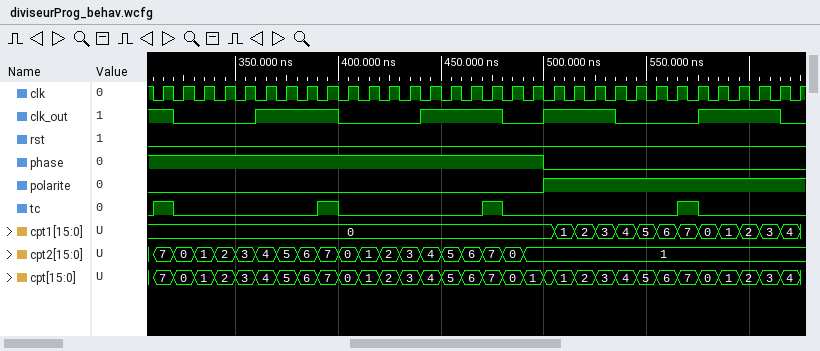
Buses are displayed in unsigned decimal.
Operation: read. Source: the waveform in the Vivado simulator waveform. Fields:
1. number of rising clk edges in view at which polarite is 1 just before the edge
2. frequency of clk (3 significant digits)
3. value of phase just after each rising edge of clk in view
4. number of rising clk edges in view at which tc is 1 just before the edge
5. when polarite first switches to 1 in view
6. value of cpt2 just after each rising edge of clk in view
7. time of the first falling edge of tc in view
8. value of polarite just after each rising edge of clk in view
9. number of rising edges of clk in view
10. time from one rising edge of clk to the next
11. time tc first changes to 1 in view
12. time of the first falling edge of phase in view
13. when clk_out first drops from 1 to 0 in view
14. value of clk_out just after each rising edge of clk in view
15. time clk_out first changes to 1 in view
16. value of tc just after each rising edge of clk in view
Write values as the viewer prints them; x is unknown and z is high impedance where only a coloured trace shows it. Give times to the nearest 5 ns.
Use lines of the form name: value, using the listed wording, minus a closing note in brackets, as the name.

number of rising clk edges in view at which polarite is 1 just before the edge: 13
frequency of clk: 100 MHz
value of phase just after each rising edge of clk in view: 1 1 1 1 1 1 1 1 1 1 1 1 1 1 1 1 1 1 1 0 0 0 0 0 0 0 0 0 0 0 0 0
number of rising clk edges in view at which tc is 1 just before the edge: 4
when polarite first switches to 1 in view: 500 ns
value of cpt2 just after each rising edge of clk in view: 7, 0, 1, 2, 3, 4, 5, 6, 7, 0, 1, 2, 3, 4, 5, 6, 7, 0, 1, 1, 1, 1, 1, 1, 1, 1, 1, 1, 1, 1, 1, 1
time of the first falling edge of tc in view: 320 ns
value of polarite just after each rising edge of clk in view: 0 0 0 0 0 0 0 0 0 0 0 0 0 0 0 0 0 0 0 1 1 1 1 1 1 1 1 1 1 1 1 1
number of rising edges of clk in view: 32
time from one rising edge of clk to the next: 10 ns
time tc first changes to 1 in view: 310 ns
time of the first falling edge of phase in view: 500 ns
when clk_out first drops from 1 to 0 in view: 320 ns
value of clk_out just after each rising edge of clk in view: 1 0 0 0 0 1 1 1 1 0 0 0 0 1 1 1 1 0 0 1 1 1 0 0 0 0 1 1 1 1 0 0
time clk_out first changes to 1 in view: 360 ns
value of tc just after each rising edge of clk in view: 1 0 0 0 0 0 0 0 1 0 0 0 0 0 0 0 1 0 0 0 0 0 0 0 0 1 0 0 0 0 0 0
